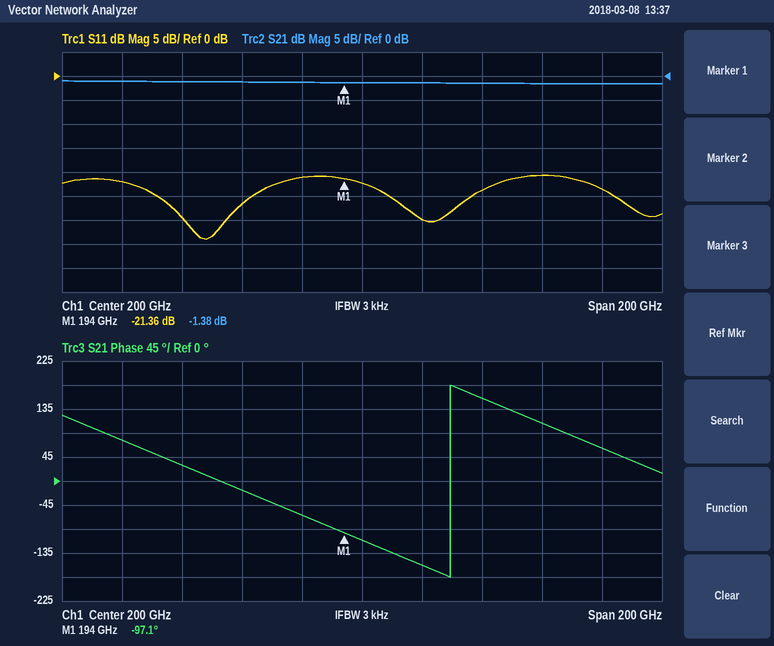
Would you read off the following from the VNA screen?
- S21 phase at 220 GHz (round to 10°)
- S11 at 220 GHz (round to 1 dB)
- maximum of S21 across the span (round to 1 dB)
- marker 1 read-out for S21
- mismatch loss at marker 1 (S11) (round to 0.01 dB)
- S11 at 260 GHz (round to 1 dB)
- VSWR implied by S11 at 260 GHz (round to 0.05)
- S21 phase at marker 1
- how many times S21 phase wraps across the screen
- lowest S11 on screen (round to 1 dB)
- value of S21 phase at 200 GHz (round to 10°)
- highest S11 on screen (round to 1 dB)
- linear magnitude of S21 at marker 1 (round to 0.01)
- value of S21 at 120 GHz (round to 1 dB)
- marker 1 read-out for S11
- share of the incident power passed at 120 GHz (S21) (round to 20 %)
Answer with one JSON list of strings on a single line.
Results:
["-160°", "-30 dB", "-1 dB", "-1.38 dB", "0.03 dB", "-21 dB", "1.20", "-97.1°", "1", "-34 dB", "-110°", "-21 dB", "0.85", "-1 dB", "-21.36 dB", "80 %"]
